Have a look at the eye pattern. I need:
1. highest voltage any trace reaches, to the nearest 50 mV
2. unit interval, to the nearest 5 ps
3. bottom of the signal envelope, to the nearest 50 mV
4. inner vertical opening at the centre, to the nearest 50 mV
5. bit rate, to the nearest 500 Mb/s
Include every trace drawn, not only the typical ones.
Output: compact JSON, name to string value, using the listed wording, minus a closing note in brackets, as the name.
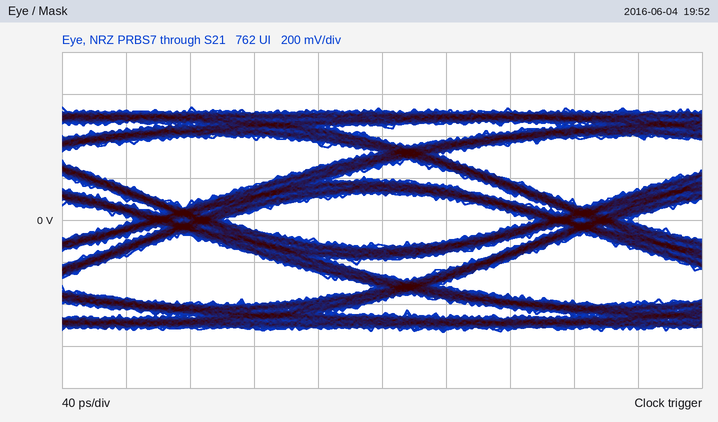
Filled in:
{"highest voltage any trace reaches, to the nearest 50 mV": "550 mV", "unit interval, to the nearest 5 ps": "250 ps", "bottom of the signal envelope, to the nearest 50 mV": "-550 mV", "inner vertical opening at the centre, to the nearest 50 mV": "250 mV", "bit rate, to the nearest 500 Mb/s": "4.0 Gb/s"}
